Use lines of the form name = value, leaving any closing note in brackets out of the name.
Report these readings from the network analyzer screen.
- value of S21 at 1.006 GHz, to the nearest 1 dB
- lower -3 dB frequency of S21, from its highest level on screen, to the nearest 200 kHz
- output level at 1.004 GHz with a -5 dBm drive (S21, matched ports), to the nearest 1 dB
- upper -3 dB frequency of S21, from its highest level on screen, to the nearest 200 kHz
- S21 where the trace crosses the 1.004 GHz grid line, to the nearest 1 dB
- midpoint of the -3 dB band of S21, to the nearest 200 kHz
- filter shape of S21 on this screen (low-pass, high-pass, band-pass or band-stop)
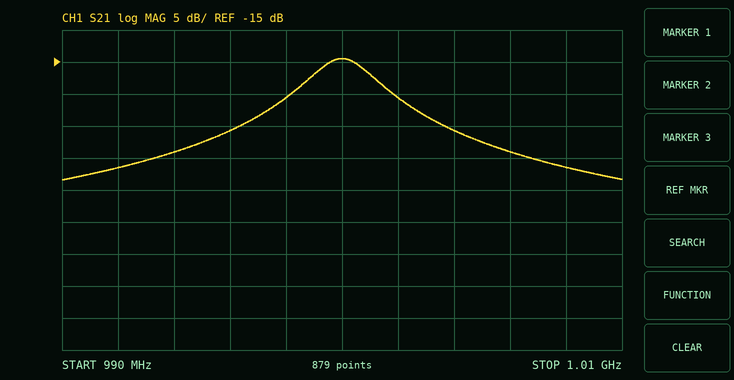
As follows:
value of S21 at 1.006 GHz, to the nearest 1 dB = -29 dB
lower -3 dB frequency of S21, from its highest level on screen, to the nearest 200 kHz = 998.8 MHz
output level at 1.004 GHz with a -5 dBm drive (S21, matched ports), to the nearest 1 dB = -31 dBm
upper -3 dB frequency of S21, from its highest level on screen, to the nearest 200 kHz = 1.0012 GHz
S21 where the trace crosses the 1.004 GHz grid line, to the nearest 1 dB = -26 dB
midpoint of the -3 dB band of S21, to the nearest 200 kHz = 1.0000 GHz
filter shape of S21 on this screen = band-pass
